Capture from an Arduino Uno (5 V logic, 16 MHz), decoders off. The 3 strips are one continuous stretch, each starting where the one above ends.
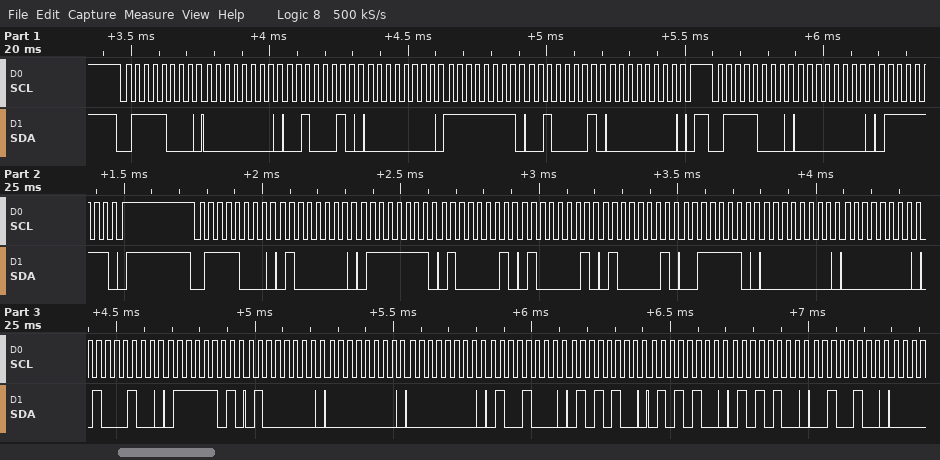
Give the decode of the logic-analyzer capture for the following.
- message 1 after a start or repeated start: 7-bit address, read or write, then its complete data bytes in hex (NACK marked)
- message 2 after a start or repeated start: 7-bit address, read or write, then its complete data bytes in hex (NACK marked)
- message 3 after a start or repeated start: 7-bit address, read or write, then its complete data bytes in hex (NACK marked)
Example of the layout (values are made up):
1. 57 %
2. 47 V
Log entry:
1. 0x3C write: 00 22 00 FF 21 00
2. 0x3C write: 00 7F
3. 0x3C write: 40 7F 41 41 41 3E 00 00 44 7D 40 00 00 48 54 54 54 24
